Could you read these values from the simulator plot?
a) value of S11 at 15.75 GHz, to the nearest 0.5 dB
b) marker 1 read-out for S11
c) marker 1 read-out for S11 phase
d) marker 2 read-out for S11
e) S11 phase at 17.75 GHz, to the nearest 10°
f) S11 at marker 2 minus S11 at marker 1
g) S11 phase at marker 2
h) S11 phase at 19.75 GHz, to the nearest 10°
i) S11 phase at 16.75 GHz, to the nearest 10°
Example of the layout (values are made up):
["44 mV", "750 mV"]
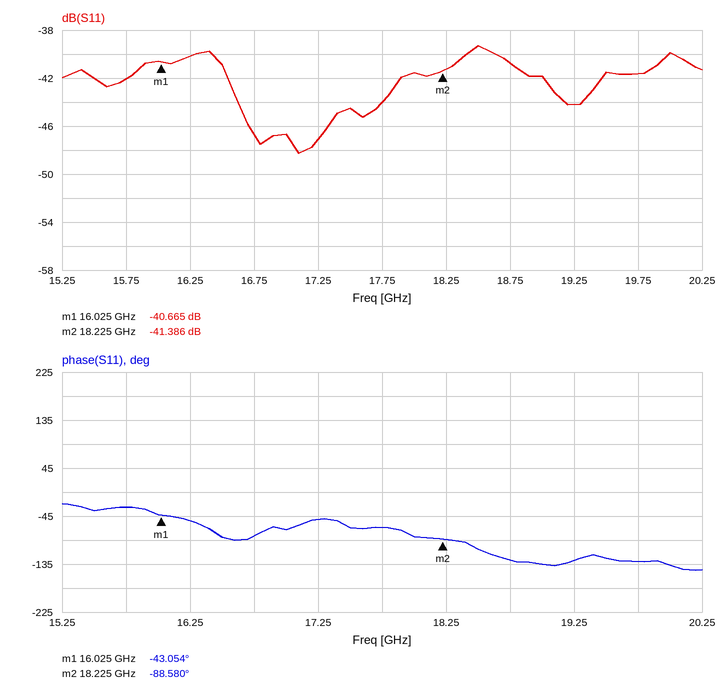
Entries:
["-42.0 dB", "-40.665 dB", "-43.054°", "-41.386 dB", "-70°", "-0.721 dB", "-88.580°", "-130°", "-80°"]
